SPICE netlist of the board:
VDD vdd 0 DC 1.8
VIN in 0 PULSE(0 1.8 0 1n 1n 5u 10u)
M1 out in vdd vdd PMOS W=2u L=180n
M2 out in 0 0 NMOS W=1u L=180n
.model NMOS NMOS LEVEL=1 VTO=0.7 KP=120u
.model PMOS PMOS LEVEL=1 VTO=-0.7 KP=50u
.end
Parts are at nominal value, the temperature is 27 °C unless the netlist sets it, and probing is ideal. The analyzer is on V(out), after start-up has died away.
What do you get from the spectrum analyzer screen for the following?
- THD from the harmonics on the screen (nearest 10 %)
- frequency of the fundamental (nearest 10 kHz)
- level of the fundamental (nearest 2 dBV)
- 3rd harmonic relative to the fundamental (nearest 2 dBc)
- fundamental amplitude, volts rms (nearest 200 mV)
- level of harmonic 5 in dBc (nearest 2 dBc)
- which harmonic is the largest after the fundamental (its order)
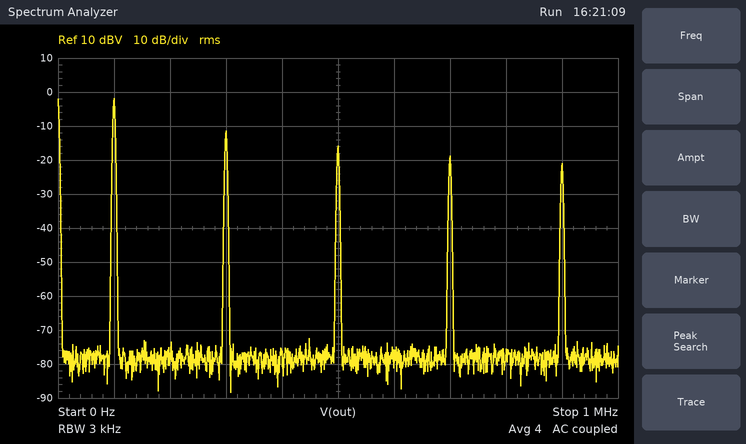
40 %
100 kHz
-2 dBV
-10 dBc
800 mV
-14 dBc
3
